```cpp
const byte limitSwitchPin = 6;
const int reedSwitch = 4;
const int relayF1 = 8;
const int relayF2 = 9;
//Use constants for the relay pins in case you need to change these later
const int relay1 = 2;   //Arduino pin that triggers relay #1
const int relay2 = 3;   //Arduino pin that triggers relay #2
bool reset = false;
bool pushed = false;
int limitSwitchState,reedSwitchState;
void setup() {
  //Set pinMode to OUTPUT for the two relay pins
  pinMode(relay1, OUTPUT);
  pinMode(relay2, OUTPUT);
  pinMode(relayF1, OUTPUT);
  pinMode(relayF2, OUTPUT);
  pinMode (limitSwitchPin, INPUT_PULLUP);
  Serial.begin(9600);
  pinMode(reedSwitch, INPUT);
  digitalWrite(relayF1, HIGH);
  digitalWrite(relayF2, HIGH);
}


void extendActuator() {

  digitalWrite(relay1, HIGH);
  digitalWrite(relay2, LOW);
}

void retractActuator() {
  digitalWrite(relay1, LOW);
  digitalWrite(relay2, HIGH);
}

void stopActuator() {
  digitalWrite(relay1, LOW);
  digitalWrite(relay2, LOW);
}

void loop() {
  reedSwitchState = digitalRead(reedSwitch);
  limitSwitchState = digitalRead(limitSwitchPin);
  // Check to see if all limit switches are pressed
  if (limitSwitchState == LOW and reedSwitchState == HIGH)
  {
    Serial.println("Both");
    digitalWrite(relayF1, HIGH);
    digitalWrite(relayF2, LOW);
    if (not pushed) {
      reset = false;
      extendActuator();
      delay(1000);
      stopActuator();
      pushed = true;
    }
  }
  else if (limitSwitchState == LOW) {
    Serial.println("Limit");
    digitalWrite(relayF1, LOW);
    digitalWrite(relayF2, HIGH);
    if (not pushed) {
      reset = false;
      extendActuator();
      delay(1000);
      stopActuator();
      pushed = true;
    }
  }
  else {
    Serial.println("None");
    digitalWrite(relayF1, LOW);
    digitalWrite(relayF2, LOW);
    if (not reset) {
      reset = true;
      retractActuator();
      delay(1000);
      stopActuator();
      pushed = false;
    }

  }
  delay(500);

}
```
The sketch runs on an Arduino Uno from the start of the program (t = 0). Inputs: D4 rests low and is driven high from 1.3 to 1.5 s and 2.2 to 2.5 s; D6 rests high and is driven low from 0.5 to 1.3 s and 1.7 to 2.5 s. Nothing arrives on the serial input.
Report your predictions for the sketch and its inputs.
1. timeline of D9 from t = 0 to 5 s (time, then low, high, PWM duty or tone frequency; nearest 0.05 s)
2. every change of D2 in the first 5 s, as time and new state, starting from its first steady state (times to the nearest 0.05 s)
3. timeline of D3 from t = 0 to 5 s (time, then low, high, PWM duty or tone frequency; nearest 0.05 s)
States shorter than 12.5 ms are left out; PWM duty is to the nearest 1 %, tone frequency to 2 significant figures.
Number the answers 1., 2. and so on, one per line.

1. 0 s low; 2 s high; 3.5 s low
2. 0 s low; 2 s high; 3 s low
3. 0 s high; 1 s low; 3.5 s high; 4.5 s low
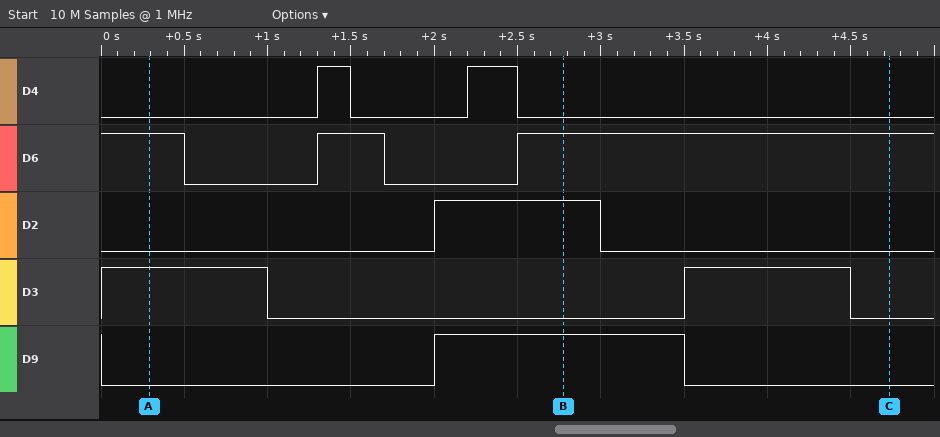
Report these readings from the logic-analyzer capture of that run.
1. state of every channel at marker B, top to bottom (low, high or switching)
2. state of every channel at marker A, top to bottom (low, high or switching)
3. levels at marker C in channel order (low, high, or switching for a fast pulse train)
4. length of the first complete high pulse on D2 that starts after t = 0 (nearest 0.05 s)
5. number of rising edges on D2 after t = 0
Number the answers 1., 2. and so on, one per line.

1. D4 low, D6 high, D2 high, D3 low, D9 high
2. D4 low, D6 high, D2 low, D3 high, D9 low
3. D4 low, D6 high, D2 low, D3 low, D9 low
4. 1.00 s
5. 1
